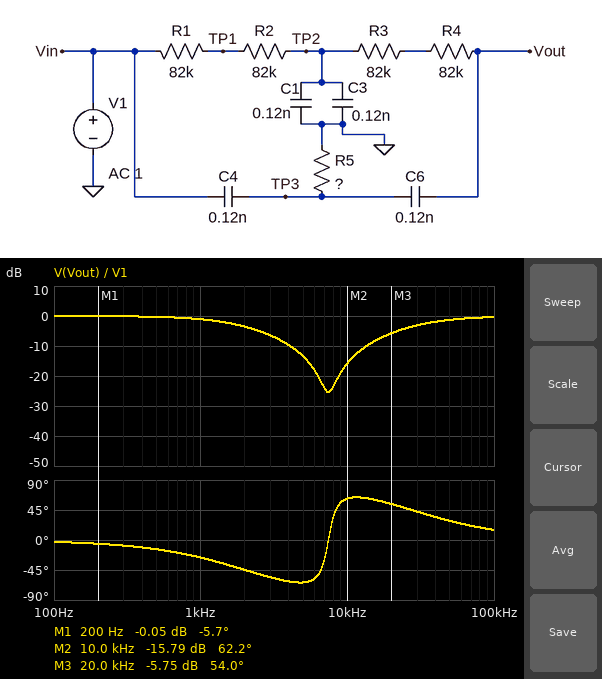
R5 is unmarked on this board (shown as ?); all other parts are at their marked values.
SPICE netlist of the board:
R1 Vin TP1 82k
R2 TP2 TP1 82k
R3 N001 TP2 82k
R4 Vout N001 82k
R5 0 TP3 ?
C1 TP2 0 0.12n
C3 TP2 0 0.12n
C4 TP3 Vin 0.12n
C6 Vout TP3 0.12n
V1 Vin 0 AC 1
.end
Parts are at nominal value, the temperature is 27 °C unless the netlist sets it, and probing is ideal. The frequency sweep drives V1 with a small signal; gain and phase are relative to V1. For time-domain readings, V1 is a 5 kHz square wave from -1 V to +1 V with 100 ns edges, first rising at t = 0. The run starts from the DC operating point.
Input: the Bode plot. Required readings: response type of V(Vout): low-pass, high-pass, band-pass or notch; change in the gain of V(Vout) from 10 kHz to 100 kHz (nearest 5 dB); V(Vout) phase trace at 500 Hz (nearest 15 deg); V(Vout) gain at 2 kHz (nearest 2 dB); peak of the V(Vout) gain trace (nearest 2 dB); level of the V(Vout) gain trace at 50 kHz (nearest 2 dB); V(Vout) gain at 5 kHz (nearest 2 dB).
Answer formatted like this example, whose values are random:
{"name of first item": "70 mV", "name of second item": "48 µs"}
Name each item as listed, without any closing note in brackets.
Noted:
{"response type of V(Vout): low-pass, high-pass, band-pass or notch": "notch", "change in the gain of V(Vout) from 10 kHz to 100 kHz": "15 dB", "V(Vout) phase trace at 500 Hz": "-15 deg", "V(Vout) gain at 2 kHz": "-4 dB", "peak of the V(Vout) gain trace": "0 dB", "level of the V(Vout) gain trace at 50 kHz": "-2 dB", "V(Vout) gain at 5 kHz": "-14 dB"}
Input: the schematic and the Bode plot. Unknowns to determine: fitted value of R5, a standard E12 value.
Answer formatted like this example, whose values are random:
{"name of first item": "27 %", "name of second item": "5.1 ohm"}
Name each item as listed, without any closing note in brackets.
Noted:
{"fitted value of R5, a standard E12 value": "120 kΩ"}
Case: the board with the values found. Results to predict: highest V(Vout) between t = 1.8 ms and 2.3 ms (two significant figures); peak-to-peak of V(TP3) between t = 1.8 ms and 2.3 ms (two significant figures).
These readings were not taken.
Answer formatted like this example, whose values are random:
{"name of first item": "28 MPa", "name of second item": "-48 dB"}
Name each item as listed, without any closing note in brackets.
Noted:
{"highest V(Vout) between t = 1.8 ms and 2.3 ms": "1.5 V", "peak-to-peak of V(TP3) between t = 1.8 ms and 2.3 ms": "3.7 V"}
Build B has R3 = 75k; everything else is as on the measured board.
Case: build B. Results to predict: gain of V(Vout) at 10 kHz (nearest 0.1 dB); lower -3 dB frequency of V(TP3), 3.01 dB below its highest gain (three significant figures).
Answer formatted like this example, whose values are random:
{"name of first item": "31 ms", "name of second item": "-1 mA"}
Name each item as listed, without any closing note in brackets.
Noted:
{"gain of V(Vout) at 10 kHz": "-16.3 dB", "lower -3 dB frequency of V(TP3), 3.01 dB below its highest gain": "23.8 kHz"}
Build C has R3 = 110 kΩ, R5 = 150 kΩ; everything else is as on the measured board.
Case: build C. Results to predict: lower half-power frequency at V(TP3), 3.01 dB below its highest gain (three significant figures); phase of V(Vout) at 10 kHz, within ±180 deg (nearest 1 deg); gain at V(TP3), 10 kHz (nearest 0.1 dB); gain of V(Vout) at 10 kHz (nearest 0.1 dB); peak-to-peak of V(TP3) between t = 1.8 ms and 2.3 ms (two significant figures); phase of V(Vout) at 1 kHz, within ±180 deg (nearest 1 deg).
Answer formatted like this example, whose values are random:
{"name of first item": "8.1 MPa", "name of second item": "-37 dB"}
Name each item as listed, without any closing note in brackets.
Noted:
{"lower half-power frequency at V(TP3), 3.01 dB below its highest gain": "19.6 kHz", "phase of V(Vout) at 10 kHz, within ±180 deg": "58 deg", "gain at V(TP3), 10 kHz": "-5.7 dB", "gain of V(Vout) at 10 kHz": "-12.7 dB", "peak-to-peak of V(TP3) between t = 1.8 ms and 2.3 ms": "3.6 V", "phase of V(Vout) at 1 kHz, within ±180 deg": "-27 deg"}
